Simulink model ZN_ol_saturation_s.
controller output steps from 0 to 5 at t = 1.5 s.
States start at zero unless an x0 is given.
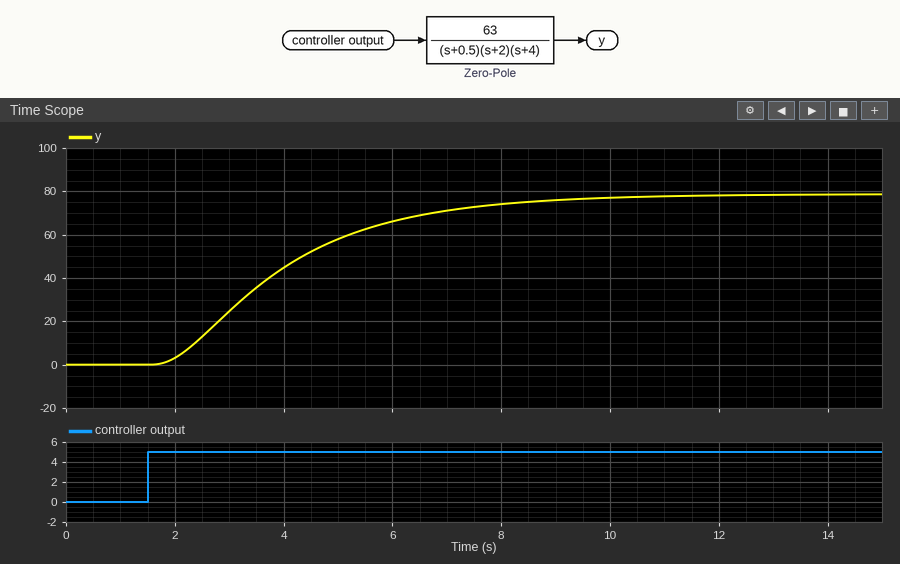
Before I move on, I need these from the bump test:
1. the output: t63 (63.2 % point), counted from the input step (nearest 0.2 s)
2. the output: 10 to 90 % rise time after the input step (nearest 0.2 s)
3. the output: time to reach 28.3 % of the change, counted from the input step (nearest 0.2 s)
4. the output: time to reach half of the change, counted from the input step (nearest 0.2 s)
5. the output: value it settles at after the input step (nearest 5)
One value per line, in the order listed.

2.8 s
4.6 s
1.4 s
2.2 s
80
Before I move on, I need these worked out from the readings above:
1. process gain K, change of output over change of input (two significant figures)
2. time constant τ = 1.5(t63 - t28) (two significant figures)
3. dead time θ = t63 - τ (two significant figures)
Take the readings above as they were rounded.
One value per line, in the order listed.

16
2.1 s
0.70 s
